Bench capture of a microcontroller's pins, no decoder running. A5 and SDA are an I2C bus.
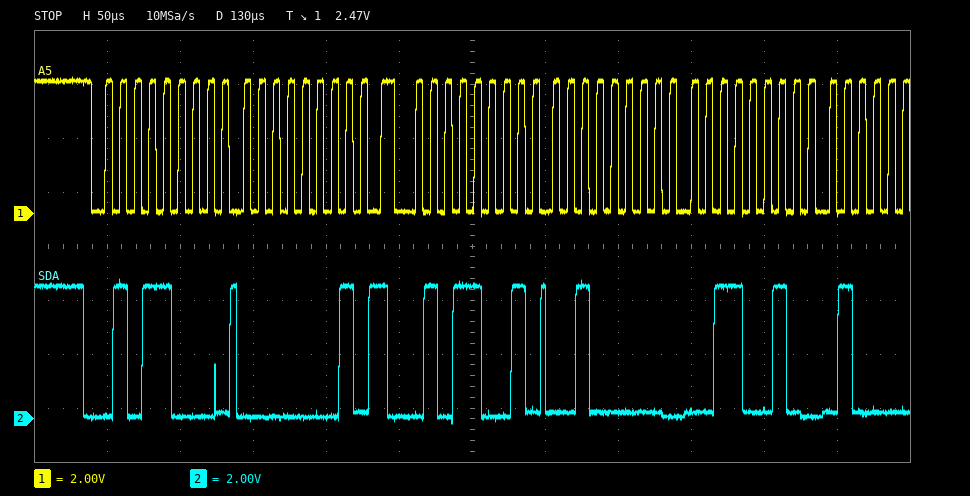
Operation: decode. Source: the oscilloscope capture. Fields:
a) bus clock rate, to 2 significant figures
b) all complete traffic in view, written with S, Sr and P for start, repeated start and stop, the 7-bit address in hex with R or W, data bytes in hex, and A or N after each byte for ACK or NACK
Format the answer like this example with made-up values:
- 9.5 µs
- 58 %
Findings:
- 100 kHz
- S 2CW A 01 A Sr 2CR A 20 A 32 A
